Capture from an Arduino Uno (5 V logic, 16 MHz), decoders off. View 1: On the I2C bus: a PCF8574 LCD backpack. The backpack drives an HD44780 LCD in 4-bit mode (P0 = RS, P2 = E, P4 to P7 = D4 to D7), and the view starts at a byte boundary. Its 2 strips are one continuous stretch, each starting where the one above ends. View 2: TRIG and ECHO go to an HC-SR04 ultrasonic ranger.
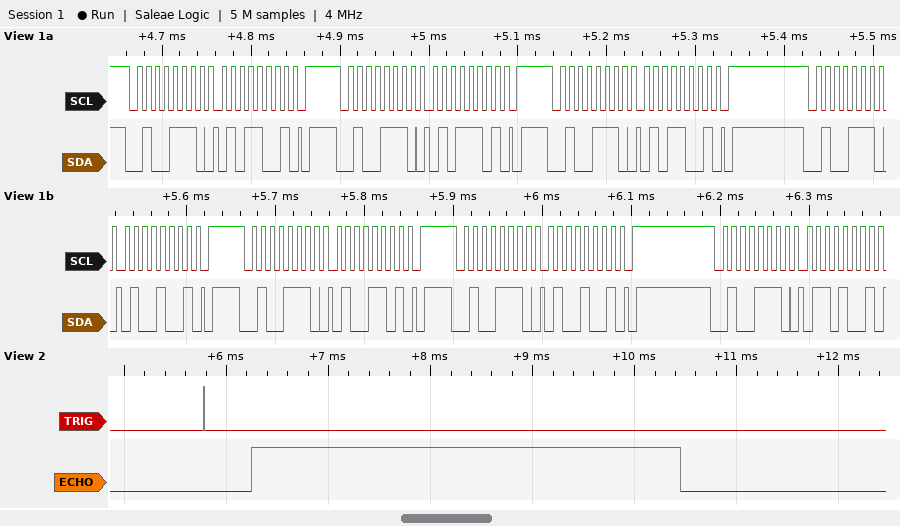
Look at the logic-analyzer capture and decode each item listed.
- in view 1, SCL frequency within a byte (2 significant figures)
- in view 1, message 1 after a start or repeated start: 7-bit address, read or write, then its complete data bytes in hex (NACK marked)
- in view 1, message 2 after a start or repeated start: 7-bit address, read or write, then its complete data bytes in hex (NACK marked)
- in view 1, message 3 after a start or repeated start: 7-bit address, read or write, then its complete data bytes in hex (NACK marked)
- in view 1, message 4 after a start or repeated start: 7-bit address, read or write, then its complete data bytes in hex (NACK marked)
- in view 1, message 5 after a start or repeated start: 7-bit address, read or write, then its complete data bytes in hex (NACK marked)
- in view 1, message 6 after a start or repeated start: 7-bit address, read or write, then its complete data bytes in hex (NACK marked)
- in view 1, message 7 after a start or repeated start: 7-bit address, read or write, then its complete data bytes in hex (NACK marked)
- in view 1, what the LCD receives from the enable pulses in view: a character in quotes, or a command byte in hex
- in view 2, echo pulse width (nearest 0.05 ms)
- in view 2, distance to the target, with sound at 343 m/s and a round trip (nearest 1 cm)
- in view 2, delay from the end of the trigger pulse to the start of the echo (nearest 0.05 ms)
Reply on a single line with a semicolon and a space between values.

100 kHz; 0x27 write: 59; 0x27 write: 5D; 0x27 write: 59; 0x27 write: 49; 0x27 write: 4D; 0x27 write: 49; 0x27 write: 69; 'T'; 4.20 ms; 72 cm; 0.45 ms
